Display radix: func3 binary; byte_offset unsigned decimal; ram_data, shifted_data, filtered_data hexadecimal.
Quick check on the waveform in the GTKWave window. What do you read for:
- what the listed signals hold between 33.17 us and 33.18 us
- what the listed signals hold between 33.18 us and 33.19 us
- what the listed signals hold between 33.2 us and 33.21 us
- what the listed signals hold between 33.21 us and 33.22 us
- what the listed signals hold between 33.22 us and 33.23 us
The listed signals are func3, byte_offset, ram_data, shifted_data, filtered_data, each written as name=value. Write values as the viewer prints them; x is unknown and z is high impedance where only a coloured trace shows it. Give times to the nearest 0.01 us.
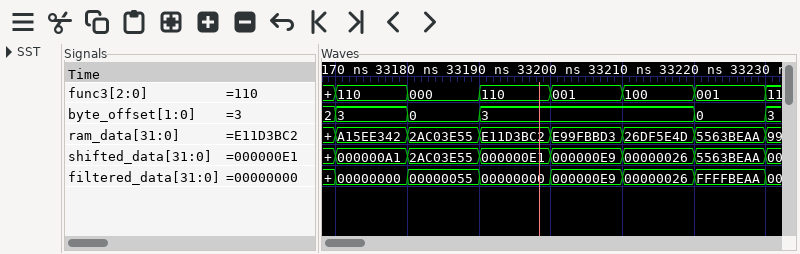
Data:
func3=110, byte_offset=3, ram_data=A15EE342, shifted_data=000000A1, filtered_data=00000000
func3=000, byte_offset=0, ram_data=2AC03E55, shifted_data=2AC03E55, filtered_data=00000055
func3=001, byte_offset=3, ram_data=E99FBBD3, shifted_data=000000E9, filtered_data=000000E9
func3=100, byte_offset=3, ram_data=26DF5E4D, shifted_data=00000026, filtered_data=00000026
func3=001, byte_offset=0, ram_data=5563BEAA, shifted_data=5563BEAA, filtered_data=FFFFBEAA
